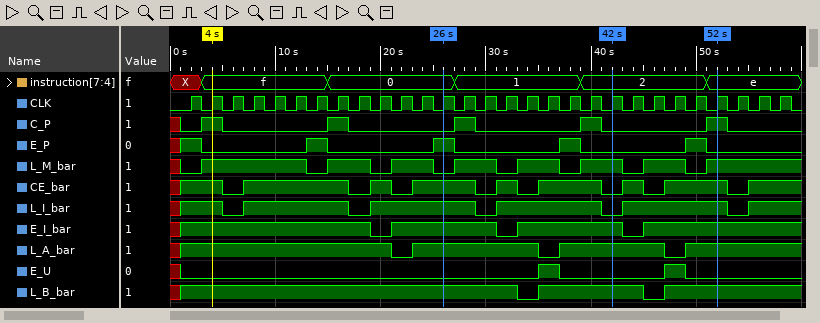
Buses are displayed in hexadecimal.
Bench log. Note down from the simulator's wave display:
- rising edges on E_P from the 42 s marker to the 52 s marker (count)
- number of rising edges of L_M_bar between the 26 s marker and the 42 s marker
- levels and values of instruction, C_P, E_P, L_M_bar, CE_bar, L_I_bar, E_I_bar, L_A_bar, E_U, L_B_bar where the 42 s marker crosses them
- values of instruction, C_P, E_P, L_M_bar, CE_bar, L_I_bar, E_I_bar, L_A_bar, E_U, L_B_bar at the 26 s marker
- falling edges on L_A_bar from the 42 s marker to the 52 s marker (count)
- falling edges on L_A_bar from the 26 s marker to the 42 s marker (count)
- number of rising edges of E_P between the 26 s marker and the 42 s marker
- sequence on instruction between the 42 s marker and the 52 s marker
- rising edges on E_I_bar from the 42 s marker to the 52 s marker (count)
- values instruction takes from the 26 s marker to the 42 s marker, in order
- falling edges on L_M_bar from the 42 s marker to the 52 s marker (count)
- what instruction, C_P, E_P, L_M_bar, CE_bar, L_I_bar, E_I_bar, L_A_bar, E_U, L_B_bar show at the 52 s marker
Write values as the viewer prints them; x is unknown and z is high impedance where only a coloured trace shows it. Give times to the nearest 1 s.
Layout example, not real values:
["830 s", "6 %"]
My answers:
["1", "3", "instruction=2, C_P=0, E_P=0, L_M_bar=1, CE_bar=0, L_I_bar=0, E_I_bar=1, L_A_bar=1, E_U=0, L_B_bar=1", "instruction=0, C_P=0, E_P=1, L_M_bar=0, CE_bar=1, L_I_bar=1, E_I_bar=1, L_A_bar=1, E_U=0, L_B_bar=1", "1", "1", "1", "2, e", "1", "0, 1, 2", "2", "instruction=e, C_P=1, E_P=0, L_M_bar=1, CE_bar=1, L_I_bar=1, E_I_bar=1, L_A_bar=1, E_U=0, L_B_bar=1"]
